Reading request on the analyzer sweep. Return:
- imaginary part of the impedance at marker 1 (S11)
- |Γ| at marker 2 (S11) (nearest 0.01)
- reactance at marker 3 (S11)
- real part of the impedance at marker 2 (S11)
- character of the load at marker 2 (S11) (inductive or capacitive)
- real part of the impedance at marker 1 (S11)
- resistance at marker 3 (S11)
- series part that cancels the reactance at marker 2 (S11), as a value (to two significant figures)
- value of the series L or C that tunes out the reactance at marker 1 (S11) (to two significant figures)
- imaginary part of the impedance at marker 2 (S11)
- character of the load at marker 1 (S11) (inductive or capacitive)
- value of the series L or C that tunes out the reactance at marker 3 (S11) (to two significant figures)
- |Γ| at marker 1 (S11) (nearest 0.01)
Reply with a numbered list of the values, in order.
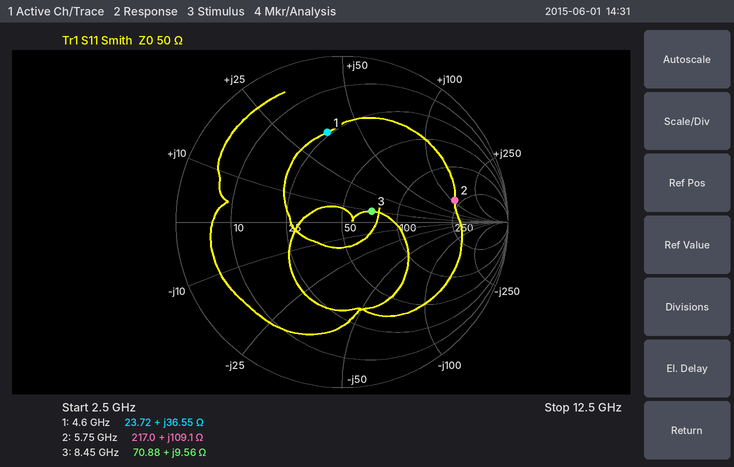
1. +36.55 Ω
2. 0.69
3. +9.56 Ω
4. 217.0 Ω
5. inductive
6. 23.72 Ω
7. 70.88 Ω
8. 250 fF
9. 950 fF
10. +109.1 Ω
11. inductive
12. 2.0 pF
13. 0.55
